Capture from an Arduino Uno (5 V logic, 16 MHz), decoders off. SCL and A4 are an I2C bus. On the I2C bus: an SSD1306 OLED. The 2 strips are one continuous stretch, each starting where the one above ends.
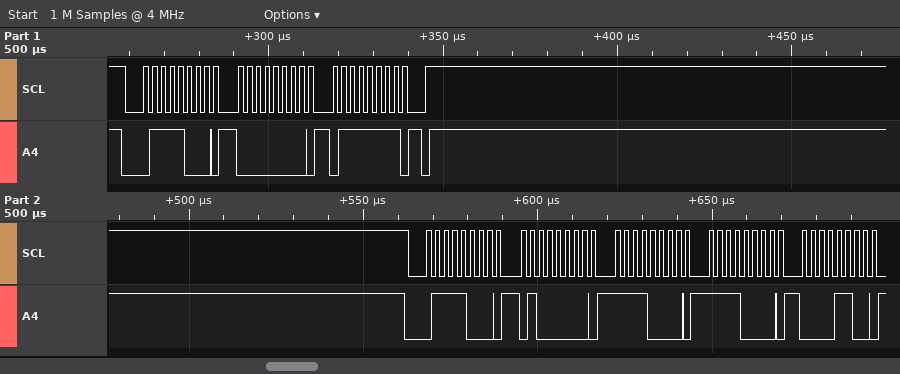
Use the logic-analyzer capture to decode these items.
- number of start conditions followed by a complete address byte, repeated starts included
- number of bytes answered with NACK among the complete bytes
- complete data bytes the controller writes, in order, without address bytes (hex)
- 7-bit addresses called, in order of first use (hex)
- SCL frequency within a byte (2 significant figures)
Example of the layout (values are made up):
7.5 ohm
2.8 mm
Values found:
2
0
00 7F 40 F0 F0 0C
0x3C
400 kHz
